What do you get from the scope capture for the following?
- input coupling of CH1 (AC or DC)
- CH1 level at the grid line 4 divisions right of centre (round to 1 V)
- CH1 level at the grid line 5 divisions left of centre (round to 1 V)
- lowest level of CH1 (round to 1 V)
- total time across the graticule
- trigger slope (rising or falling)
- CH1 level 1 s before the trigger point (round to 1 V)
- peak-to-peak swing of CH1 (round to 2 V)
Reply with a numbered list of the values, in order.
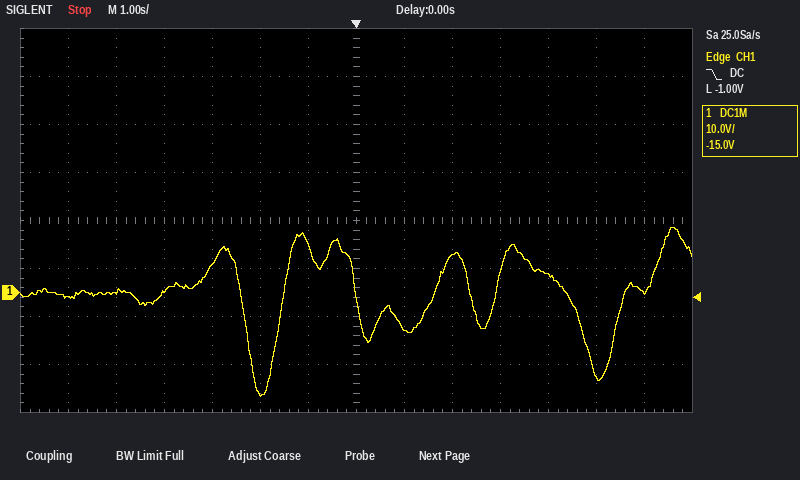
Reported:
1. DC
2. 4 V
3. 0 V
4. -22 V
5. 14 s
6. falling
7. 10 V
8. 36 V
